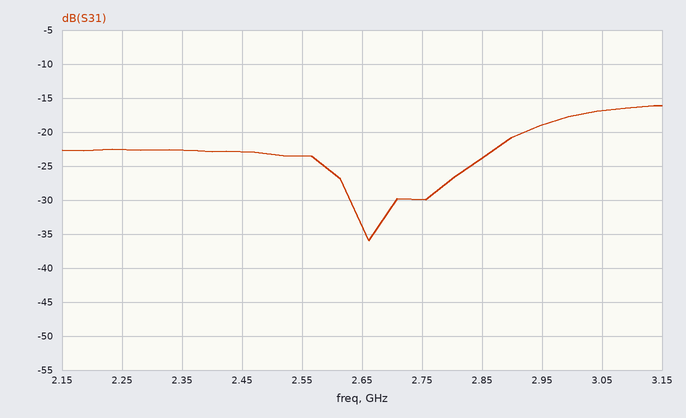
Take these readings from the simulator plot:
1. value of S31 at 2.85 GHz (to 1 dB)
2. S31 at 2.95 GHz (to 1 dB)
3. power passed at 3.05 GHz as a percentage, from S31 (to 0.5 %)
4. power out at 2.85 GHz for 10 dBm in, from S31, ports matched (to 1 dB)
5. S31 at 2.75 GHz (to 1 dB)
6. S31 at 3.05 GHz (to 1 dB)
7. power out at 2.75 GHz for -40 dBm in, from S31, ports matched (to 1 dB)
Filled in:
-24 dB
-19 dB
2.0 %
-14 dBm
-30 dB
-17 dB
-70 dBm
